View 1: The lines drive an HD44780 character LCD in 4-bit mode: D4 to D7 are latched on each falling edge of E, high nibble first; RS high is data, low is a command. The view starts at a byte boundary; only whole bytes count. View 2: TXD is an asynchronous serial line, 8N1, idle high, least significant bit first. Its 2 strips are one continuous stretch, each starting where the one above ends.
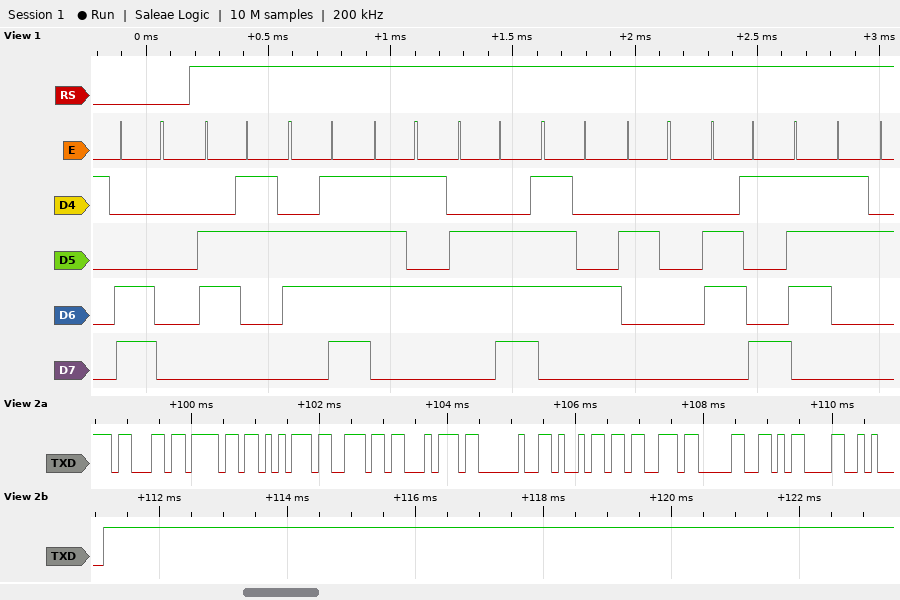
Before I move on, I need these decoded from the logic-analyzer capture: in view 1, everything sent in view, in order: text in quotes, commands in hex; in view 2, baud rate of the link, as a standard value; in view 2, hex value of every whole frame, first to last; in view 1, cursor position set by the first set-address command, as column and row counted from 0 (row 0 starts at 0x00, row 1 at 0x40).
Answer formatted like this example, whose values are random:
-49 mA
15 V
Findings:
0xC0 "count is"
9600 baud
63 6F 75 6E 74 20 69 73 30 0D 0A
column 0, row 1
